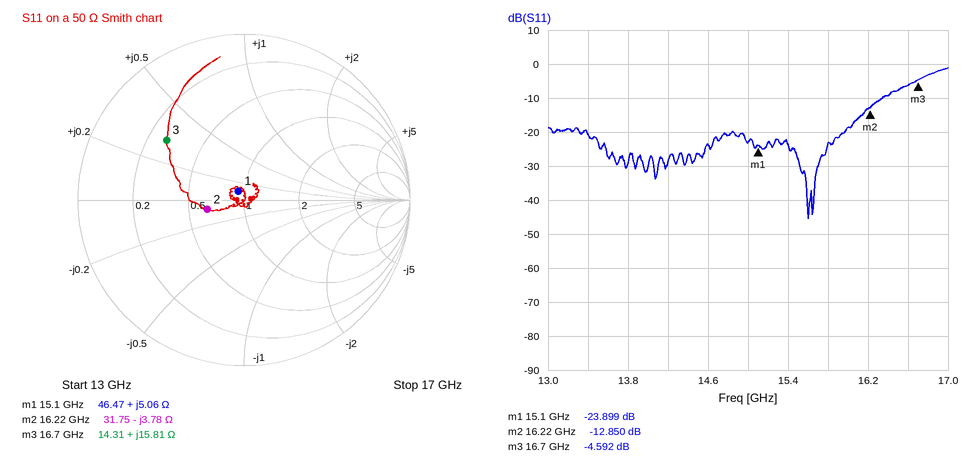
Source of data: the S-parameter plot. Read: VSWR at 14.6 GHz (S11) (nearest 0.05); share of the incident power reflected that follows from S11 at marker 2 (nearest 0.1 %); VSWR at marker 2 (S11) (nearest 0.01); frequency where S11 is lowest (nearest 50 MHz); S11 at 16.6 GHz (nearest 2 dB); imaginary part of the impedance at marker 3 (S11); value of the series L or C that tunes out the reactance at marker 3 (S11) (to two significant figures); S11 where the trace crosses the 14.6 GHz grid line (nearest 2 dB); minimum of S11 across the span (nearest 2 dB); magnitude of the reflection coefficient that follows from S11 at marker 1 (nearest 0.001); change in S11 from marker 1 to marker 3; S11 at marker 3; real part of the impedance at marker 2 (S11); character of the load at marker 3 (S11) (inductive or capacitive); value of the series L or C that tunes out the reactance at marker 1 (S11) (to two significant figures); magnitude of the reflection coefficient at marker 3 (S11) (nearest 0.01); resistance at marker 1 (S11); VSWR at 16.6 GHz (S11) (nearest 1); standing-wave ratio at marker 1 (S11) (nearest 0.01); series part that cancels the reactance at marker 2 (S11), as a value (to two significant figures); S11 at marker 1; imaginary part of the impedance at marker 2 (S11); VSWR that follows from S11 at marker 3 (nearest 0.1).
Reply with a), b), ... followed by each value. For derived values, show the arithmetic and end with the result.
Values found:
a) |Γ| = 10^(-24/20) = 0.0631; VSWR = (1 + 0.0631)/(1 − 0.0631) ≈ 1.13, so 1.15 to the nearest 0.05
b) 10^(-12.85/10) ≈ 5.2 %
c) 1.59
d) 15.60 GHz
e) -6 dB
f) +15.81 Ω
g) C = 1/(2π × 16.7 GHz × 15.81 Ω) ≈ 603 fF, so 600 fF to two significant figures
h) -24 dB
i) -46 dB
j) 10^(-23.899/20) ≈ 0.064
k) -4.592 − (-23.899) = 19.307 dB
l) -4.592 dB
m) 31.75 Ω
n) inductive
o) C = 1/(2π × 15.1 GHz × 5.06 Ω) ≈ 2.1 pF
p) 0.59
q) 46.47 Ω
r) |Γ| = 10^(-6/20) = 0.5012; VSWR = (1 + 0.5012)/(1 − 0.5012) ≈ 3
s) 1.14
t) L = 3.78 Ω/(2π × 16.22 GHz) ≈ 37 pH
u) -23.899 dB
v) -3.78 Ω
w) (1 + 0.5894)/(1 − 0.5894) ≈ 3.9
